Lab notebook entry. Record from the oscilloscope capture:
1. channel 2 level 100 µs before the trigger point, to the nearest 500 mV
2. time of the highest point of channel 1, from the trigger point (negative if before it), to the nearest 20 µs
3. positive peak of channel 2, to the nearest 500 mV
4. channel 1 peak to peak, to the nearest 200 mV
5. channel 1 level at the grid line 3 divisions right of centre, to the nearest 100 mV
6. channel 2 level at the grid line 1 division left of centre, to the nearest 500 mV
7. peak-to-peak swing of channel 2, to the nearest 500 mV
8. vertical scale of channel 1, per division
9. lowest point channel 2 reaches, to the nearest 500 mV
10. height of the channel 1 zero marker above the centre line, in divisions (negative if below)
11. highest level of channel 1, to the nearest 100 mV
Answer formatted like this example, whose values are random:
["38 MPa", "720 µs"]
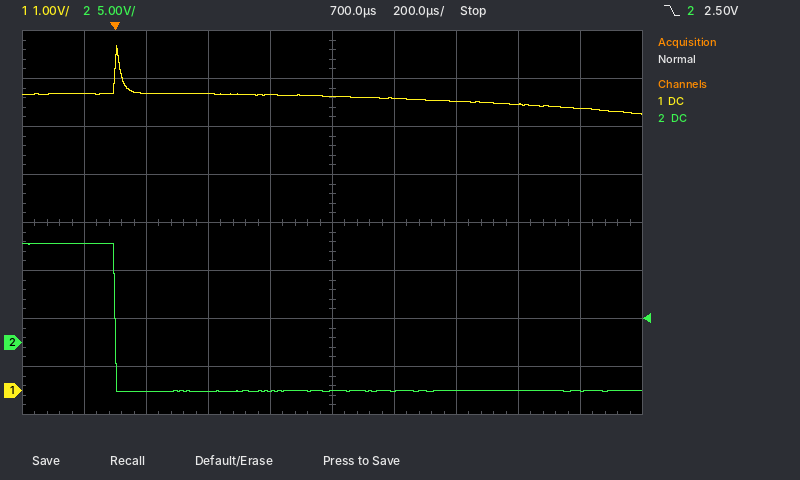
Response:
["10.5 V", "0 µs", "10.5 V", "1.4 V", "6.0 V", "-5.0 V", "15.5 V", "1 V", "-5.0 V", "-3.5 div", "7.2 V"]
